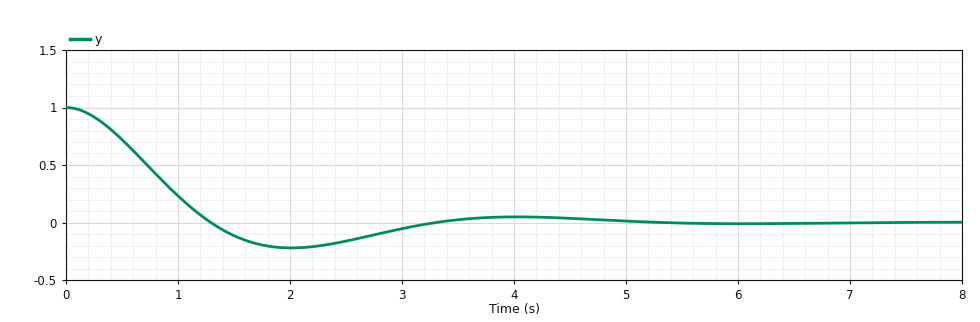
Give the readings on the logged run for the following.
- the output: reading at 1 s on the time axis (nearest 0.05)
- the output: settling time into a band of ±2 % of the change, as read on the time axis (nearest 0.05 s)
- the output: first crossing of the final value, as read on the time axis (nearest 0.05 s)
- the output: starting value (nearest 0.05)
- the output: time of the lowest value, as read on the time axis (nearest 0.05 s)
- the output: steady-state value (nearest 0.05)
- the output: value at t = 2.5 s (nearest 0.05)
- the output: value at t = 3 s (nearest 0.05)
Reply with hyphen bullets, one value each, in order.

- 0.25
- 4.85 s
- 1.30 s
- 1.00
- 2.00 s
- 0.00
- -0.15
- -0.05
